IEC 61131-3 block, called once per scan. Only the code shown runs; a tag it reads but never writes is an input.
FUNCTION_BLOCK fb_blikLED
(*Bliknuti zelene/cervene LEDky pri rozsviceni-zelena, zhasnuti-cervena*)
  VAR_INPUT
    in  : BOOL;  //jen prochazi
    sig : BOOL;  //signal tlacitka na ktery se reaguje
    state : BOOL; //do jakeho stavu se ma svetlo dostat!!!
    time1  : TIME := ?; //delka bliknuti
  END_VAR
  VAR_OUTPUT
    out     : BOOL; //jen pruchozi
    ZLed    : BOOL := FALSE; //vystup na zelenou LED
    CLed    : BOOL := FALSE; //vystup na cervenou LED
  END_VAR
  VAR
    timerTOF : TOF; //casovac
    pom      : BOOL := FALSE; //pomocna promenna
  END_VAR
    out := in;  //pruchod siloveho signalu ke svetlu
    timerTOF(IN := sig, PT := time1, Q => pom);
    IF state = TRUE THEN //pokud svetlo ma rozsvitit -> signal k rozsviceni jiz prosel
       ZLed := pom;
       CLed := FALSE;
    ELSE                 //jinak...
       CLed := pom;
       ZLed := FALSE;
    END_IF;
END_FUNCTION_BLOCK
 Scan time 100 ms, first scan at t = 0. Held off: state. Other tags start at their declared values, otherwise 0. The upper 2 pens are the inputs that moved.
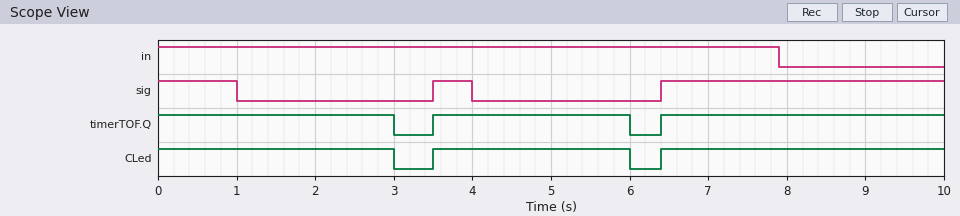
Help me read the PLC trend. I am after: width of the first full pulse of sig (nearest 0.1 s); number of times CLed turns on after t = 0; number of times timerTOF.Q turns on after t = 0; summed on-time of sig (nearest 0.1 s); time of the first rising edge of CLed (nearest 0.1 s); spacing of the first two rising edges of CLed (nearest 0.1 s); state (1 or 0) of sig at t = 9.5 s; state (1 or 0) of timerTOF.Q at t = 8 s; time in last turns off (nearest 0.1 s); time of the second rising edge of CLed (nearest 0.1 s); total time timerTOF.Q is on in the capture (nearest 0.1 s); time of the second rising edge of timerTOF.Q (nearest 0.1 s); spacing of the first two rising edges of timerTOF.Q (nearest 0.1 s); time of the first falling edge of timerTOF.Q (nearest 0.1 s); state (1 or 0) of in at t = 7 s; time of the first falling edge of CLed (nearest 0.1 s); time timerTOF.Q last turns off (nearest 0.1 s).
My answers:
0.5 s
2
2
5.1 s
3.5 s
2.9 s
1
1
7.9 s
6.4 s
9.1 s
6.4 s
2.9 s
3.0 s
1
3.0 s
6.0 s
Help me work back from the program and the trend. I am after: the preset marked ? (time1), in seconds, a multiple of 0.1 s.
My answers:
2.0 s
